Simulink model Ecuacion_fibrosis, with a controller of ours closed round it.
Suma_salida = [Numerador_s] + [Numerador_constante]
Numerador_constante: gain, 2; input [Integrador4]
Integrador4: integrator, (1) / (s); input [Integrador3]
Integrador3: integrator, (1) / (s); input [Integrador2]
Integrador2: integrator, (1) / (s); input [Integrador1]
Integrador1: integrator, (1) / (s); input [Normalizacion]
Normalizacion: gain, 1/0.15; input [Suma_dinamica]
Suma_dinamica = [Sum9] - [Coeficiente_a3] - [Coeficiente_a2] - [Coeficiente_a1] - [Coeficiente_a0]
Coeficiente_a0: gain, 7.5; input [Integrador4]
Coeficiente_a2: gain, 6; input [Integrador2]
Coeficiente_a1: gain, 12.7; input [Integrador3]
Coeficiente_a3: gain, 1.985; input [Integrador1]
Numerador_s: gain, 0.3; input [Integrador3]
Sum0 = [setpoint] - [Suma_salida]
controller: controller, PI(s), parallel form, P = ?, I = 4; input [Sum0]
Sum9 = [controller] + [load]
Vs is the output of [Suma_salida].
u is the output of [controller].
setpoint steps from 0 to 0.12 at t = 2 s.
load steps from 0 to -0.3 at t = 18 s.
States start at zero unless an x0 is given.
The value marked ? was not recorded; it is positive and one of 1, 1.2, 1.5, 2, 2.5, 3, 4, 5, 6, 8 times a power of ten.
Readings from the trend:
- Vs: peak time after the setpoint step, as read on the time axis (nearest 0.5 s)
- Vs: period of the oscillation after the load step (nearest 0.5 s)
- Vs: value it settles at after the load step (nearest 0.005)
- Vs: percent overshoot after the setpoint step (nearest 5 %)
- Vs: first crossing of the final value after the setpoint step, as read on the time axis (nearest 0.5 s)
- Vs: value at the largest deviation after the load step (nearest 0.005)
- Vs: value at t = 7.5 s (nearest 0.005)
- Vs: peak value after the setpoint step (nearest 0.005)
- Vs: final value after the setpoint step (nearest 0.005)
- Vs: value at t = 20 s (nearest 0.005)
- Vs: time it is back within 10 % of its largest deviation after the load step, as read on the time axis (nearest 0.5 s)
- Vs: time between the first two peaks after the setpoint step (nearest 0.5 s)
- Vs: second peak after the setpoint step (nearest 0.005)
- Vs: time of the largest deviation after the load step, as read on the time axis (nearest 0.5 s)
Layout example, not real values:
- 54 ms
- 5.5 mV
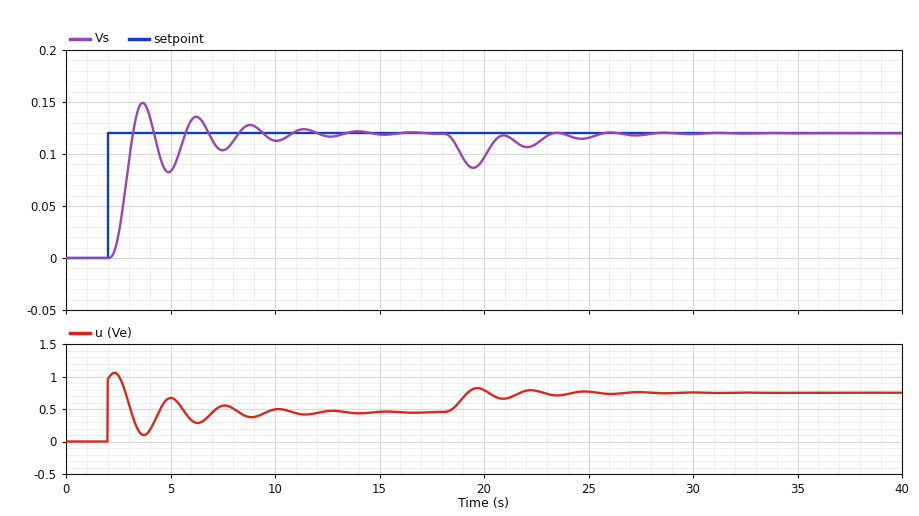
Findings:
- 3.5 s
- 2.5 s
- 0.120
- 25 %
- 3.0 s
- 0.085
- 0.105
- 0.150
- 0.120
- 0.095
- 25.0 s
- 2.5 s
- 0.135
- 19.5 s
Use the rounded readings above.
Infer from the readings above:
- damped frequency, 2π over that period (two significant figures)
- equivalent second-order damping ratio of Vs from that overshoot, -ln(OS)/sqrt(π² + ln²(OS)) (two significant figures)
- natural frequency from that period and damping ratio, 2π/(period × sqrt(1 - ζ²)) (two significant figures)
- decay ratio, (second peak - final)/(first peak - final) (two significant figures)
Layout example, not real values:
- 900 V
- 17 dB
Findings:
- 2.5 rad/s
- 0.40
- 2.7 rad/s
- 0.50
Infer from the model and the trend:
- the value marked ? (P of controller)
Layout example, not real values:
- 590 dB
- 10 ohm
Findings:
- 8
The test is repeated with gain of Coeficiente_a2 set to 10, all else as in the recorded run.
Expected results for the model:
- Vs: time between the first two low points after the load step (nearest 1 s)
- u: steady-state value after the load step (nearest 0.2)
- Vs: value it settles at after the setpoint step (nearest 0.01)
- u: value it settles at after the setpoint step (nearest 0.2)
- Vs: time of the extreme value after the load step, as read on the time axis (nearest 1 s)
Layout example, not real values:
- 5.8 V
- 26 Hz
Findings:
- 4 s
- 0.8
- 0.12
- 0.4
- 20 s
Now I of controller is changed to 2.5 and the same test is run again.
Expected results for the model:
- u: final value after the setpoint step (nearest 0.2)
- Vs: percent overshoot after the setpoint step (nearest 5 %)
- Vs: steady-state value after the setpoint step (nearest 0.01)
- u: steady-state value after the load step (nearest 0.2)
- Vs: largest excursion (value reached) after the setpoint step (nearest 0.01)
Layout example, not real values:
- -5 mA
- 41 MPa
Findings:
- 0.4
- 15 %
- 0.12
- 0.8
- 0.14
